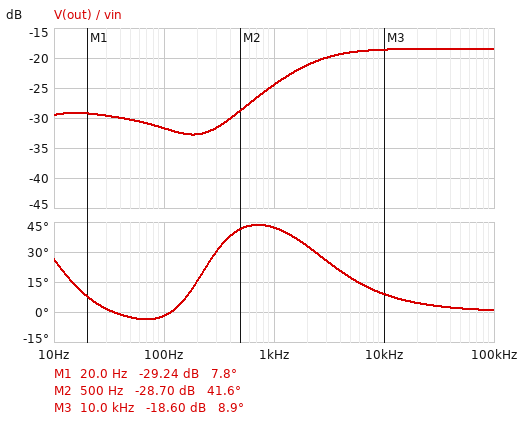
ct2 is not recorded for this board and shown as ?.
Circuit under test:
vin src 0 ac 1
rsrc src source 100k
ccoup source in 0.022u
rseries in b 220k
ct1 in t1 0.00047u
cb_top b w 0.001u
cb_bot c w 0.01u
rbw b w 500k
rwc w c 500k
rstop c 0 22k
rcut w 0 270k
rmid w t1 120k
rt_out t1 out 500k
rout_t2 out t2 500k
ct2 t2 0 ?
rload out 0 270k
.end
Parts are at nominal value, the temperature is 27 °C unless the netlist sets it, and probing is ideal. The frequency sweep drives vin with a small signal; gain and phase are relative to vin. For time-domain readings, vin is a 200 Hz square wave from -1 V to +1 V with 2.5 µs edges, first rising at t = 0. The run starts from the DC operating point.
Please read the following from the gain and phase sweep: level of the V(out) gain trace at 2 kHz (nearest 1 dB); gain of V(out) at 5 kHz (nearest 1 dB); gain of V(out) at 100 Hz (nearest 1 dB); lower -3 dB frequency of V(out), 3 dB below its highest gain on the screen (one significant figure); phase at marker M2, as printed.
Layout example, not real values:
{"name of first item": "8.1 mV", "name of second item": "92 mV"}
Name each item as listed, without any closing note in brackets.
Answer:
{"level of the V(out) gain trace at 2 kHz": "-21 dB", "gain of V(out) at 5 kHz": "-19 dB", "gain of V(out) at 100 Hz": "-32 dB", "lower -3 dB frequency of V(out), 3 dB below its highest gain on the screen": "2 kHz", "phase at marker M2, as printed": "41.6 deg"}
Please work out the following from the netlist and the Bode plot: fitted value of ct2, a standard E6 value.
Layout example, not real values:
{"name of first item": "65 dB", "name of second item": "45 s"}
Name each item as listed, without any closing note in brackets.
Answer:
{"fitted value of ct2, a standard E6 value": "15 nF"}
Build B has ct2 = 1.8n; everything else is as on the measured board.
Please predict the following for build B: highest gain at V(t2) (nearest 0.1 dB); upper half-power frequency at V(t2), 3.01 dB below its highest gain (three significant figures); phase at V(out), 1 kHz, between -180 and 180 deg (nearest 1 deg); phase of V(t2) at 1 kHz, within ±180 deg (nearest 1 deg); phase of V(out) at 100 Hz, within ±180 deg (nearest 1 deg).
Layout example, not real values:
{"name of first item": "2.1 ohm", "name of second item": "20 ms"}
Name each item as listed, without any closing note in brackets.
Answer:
{"highest gain at V(t2)": "-27.7 dB", "upper half-power frequency at V(t2), 3.01 dB below its highest gain": "93.2 Hz", "phase at V(out), 1 kHz, between -180 and 180 deg": "40 deg", "phase of V(t2) at 1 kHz, within ±180 deg": "-40 deg", "phase of V(out) at 100 Hz, within ±180 deg": "-8 deg"}
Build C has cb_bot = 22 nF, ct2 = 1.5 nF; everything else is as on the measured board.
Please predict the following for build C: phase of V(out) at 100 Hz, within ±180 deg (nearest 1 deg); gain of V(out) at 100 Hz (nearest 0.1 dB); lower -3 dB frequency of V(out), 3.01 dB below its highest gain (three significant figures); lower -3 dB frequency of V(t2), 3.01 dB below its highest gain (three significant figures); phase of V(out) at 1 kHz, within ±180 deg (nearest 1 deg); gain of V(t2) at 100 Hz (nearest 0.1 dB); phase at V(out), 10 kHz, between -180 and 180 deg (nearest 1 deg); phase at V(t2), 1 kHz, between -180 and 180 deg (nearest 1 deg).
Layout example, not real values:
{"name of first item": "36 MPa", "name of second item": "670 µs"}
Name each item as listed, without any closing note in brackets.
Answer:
{"phase of V(out) at 100 Hz, within ±180 deg": "-10 deg", "gain of V(out) at 100 Hz": "-34.1 dB", "lower -3 dB frequency of V(out), 3.01 dB below its highest gain": "1.82 kHz", "lower -3 dB frequency of V(t2), 3.01 dB below its highest gain": "5.63 Hz", "phase of V(out) at 1 kHz, within ±180 deg": "43 deg", "gain of V(t2) at 100 Hz": "-35.0 dB", "phase at V(out), 10 kHz, between -180 and 180 deg": "9 deg", "phase at V(t2), 1 kHz, between -180 and 180 deg": "-35 deg"}
